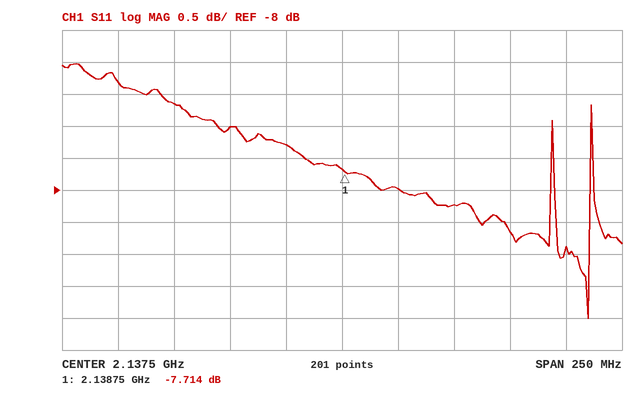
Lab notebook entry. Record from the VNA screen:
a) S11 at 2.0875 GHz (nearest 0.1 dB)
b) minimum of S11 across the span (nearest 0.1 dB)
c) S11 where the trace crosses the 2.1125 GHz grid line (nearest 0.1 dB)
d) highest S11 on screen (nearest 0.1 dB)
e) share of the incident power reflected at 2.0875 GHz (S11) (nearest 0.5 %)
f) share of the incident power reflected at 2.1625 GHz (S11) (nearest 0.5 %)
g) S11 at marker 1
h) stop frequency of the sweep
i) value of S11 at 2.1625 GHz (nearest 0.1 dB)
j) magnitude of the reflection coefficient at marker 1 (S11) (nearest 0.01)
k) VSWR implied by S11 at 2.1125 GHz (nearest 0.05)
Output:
-7.0 dB
-10.0 dB
-7.3 dB
-6.0 dB
20.0 %
16.0 %
-7.714 dB
2.2625 GHz
-8.0 dB
0.41
2.50
